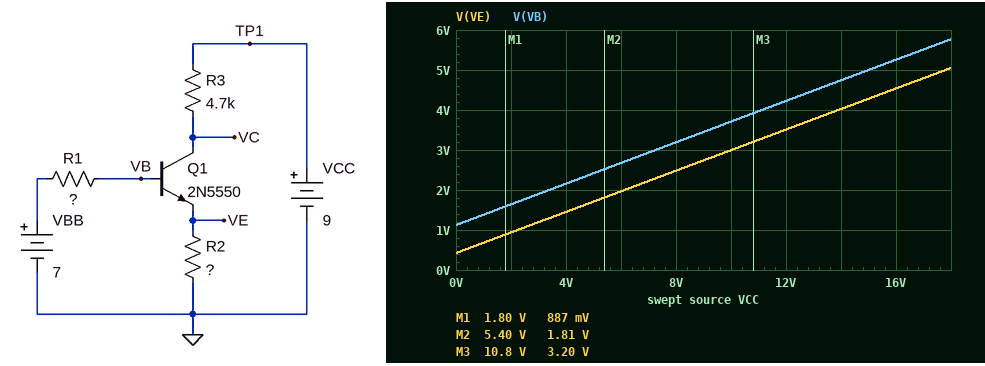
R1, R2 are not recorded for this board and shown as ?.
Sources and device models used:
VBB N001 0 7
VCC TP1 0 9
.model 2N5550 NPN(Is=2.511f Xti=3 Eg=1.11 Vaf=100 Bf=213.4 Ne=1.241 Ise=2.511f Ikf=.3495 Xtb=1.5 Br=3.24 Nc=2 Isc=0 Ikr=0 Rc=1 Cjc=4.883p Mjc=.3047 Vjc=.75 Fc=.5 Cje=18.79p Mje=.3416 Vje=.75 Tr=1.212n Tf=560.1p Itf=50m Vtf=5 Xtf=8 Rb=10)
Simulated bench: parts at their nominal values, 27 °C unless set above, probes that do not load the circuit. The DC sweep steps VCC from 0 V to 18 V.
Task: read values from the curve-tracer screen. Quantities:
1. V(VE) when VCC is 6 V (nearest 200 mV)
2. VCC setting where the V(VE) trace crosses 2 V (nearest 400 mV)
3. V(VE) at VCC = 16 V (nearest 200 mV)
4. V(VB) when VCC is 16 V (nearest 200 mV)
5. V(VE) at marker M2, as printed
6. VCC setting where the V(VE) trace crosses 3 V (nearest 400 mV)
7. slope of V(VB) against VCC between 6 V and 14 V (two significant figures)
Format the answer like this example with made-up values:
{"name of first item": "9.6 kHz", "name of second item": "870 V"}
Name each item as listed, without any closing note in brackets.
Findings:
{"V(VE) when VCC is 6 V": "2.0 V", "VCC setting where the V(VE) trace crosses 2 V": "6.0 V", "V(VE) at VCC = 16 V": "4.6 V", "V(VB) when VCC is 16 V": "5.2 V", "V(VE) at marker M2, as printed": "1.81 V", "VCC setting where the V(VE) trace crosses 3 V": "10.0 V", "slope of V(VB) against VCC between 6 V and 14 V": "0.26 V/V"}
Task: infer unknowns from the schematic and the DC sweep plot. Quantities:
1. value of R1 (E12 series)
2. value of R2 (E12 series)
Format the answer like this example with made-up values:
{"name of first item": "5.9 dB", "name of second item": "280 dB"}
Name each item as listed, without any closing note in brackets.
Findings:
{"value of R1": "18 kΩ", "value of R2": "1.8 kΩ"}
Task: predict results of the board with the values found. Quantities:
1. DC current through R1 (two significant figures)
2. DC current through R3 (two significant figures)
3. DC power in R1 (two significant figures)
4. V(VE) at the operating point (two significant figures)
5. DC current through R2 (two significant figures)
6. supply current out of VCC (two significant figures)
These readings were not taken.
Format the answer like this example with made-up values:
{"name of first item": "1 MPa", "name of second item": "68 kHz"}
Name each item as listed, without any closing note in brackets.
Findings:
{"DC current through R1": "200 µA", "DC current through R3": "1.3 mA", "DC power in R1": "700 µW", "V(VE) at the operating point": "2.7 V", "DC current through R2": "1.5 mA", "supply current out of VCC": "1.3 mA"}
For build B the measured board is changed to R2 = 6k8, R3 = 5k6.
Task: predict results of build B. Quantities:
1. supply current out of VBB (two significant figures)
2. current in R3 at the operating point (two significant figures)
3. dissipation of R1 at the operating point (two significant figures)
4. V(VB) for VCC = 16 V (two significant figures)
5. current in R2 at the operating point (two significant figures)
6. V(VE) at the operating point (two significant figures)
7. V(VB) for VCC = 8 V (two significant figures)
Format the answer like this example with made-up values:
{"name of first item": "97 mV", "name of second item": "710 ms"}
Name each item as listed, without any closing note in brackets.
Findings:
{"supply current out of VBB": "66 µA", "current in R3 at the operating point": "690 µA", "dissipation of R1 at the operating point": "79 µW", "V(VB) for VCC = 16 V": "6.8 V", "current in R2 at the operating point": "750 µA", "V(VE) at the operating point": "5.1 V", "V(VB) for VCC = 8 V": "5.3 V"}
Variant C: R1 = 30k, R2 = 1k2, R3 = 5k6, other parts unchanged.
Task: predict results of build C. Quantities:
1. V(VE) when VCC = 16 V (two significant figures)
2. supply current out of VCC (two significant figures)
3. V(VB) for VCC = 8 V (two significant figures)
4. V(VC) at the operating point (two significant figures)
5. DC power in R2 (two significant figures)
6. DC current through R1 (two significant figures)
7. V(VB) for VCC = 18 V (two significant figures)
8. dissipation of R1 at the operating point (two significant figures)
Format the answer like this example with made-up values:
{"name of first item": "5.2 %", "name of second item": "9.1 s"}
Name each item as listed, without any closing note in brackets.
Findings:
{"V(VE) when VCC = 16 V": "2.9 V", "supply current out of VCC": "1.3 mA", "V(VB) for VCC = 8 V": "2.3 V", "V(VC) at the operating point": "1.8 V", "DC power in R2": "2.5 mW", "DC current through R1": "150 µA", "V(VB) for VCC = 18 V": "4.0 V", "dissipation of R1 at the operating point": "690 µW"}
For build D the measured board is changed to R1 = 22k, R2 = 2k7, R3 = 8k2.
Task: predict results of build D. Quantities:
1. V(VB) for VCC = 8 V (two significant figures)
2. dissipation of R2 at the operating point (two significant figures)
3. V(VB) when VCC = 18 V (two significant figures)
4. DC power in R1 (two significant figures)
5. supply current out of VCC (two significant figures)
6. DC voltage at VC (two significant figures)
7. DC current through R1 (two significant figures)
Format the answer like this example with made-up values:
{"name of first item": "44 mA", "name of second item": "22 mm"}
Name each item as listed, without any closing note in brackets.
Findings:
{"V(VB) for VCC = 8 V": "3.0 V", "dissipation of R2 at the operating point": "2.4 mW", "V(VB) when VCC = 18 V": "5.3 V", "DC power in R1": "630 µW", "supply current out of VCC": "780 µA", "DC voltage at VC": "2.6 V", "DC current through R1": "170 µA"}
